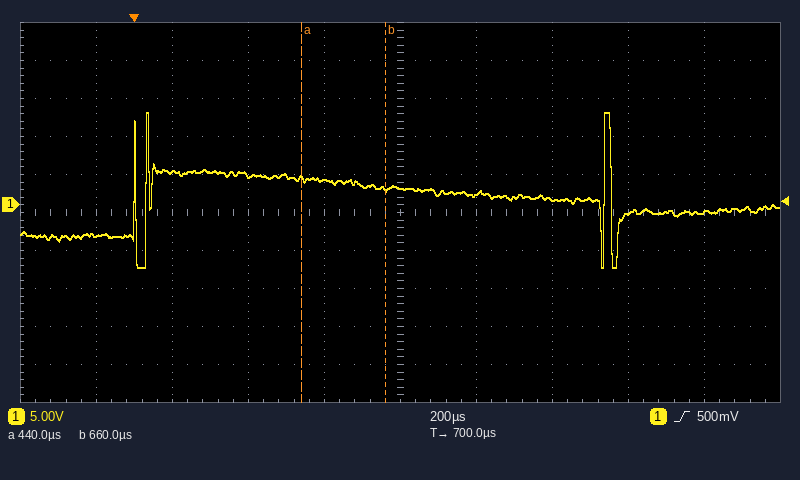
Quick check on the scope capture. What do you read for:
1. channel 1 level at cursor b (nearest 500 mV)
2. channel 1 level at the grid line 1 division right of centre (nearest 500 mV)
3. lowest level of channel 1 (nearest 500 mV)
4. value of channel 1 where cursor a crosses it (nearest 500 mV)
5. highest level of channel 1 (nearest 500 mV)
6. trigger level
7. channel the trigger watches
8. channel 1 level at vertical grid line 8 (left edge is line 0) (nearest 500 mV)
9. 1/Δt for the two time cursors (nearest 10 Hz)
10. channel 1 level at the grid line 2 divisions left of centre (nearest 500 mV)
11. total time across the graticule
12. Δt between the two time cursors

2.0 V
1.5 V
-8.0 V
3.5 V
12.0 V
500 mV
channel 1
-1.0 V
4.55 kHz
4.0 V
2 ms
220 µs
